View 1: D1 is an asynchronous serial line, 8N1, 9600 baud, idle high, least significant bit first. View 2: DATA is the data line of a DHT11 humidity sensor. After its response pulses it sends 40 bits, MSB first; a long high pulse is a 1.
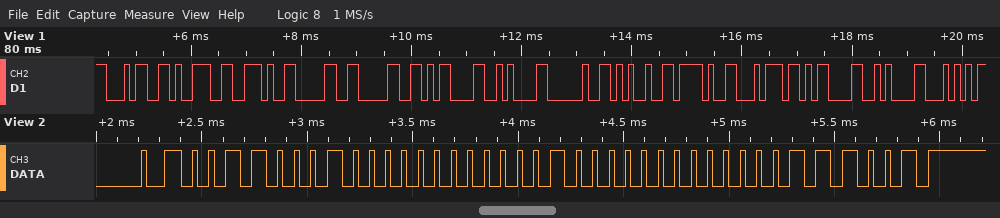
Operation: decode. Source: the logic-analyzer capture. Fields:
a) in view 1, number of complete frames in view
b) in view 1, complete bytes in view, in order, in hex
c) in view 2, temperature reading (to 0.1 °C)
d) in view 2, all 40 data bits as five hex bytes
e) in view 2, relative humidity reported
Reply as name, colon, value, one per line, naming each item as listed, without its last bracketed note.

in view 1, number of complete frames in view: 14
in view 1, complete bytes in view, in order, in hex: 34 39 2E 30 30 0D 0A 20 25 2F 74 0D 0A 54
in view 2, temperature reading: 8.0 °C
in view 2, all 40 data bits as five hex bytes: 31 00 08 00 39
in view 2, relative humidity reported: 49 %
